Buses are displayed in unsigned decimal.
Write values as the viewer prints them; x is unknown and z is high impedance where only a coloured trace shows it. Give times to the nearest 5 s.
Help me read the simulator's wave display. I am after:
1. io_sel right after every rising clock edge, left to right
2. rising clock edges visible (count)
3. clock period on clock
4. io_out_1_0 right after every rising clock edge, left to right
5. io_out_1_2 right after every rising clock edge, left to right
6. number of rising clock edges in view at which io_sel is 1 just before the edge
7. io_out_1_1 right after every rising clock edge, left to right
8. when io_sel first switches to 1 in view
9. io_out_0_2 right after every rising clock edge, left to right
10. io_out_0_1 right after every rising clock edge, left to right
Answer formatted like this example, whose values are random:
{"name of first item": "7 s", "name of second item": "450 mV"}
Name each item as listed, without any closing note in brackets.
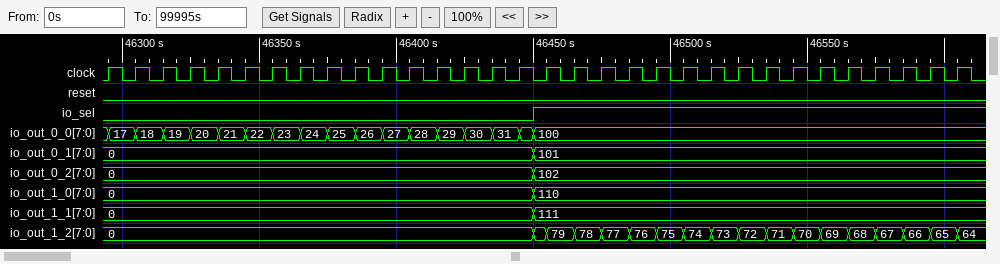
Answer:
{"io_sel right after every rising clock edge, left to right": "0 0 0 0 0 0 0 0 0 0 0 0 0 0 0 0 1 1 1 1 1 1 1 1 1 1 1 1 1 1 1 1", "rising clock edges visible": "32", "clock period on clock": "10 s", "io_out_1_0 right after every rising clock edge, left to right": "0, 0, 0, 0, 0, 0, 0, 0, 0, 0, 0, 0, 0, 0, 0, 0, 110, 110, 110, 110, 110, 110, 110, 110, 110, 110, 110, 110, 110, 110, 110, 110", "io_out_1_2 right after every rising clock edge, left to right": "0, 0, 0, 0, 0, 0, 0, 0, 0, 0, 0, 0, 0, 0, 0, 0, 79, 78, 77, 76, 75, 74, 73, 72, 71, 70, 69, 68, 67, 66, 65, 64", "number of rising clock edges in view at which io_sel is 1 just before the edge": "16", "io_out_1_1 right after every rising clock edge, left to right": "0, 0, 0, 0, 0, 0, 0, 0, 0, 0, 0, 0, 0, 0, 0, 0, 111, 111, 111, 111, 111, 111, 111, 111, 111, 111, 111, 111, 111, 111, 111, 111", "when io_sel first switches to 1 in view": "46450 s", "io_out_0_2 right after every rising clock edge, left to right": "0, 0, 0, 0, 0, 0, 0, 0, 0, 0, 0, 0, 0, 0, 0, 0, 102, 102, 102, 102, 102, 102, 102, 102, 102, 102, 102, 102, 102, 102, 102, 102", "io_out_0_1 right after every rising clock edge, left to right": "0, 0, 0, 0, 0, 0, 0, 0, 0, 0, 0, 0, 0, 0, 0, 0, 101, 101, 101, 101, 101, 101, 101, 101, 101, 101, 101, 101, 101, 101, 101, 101"}
